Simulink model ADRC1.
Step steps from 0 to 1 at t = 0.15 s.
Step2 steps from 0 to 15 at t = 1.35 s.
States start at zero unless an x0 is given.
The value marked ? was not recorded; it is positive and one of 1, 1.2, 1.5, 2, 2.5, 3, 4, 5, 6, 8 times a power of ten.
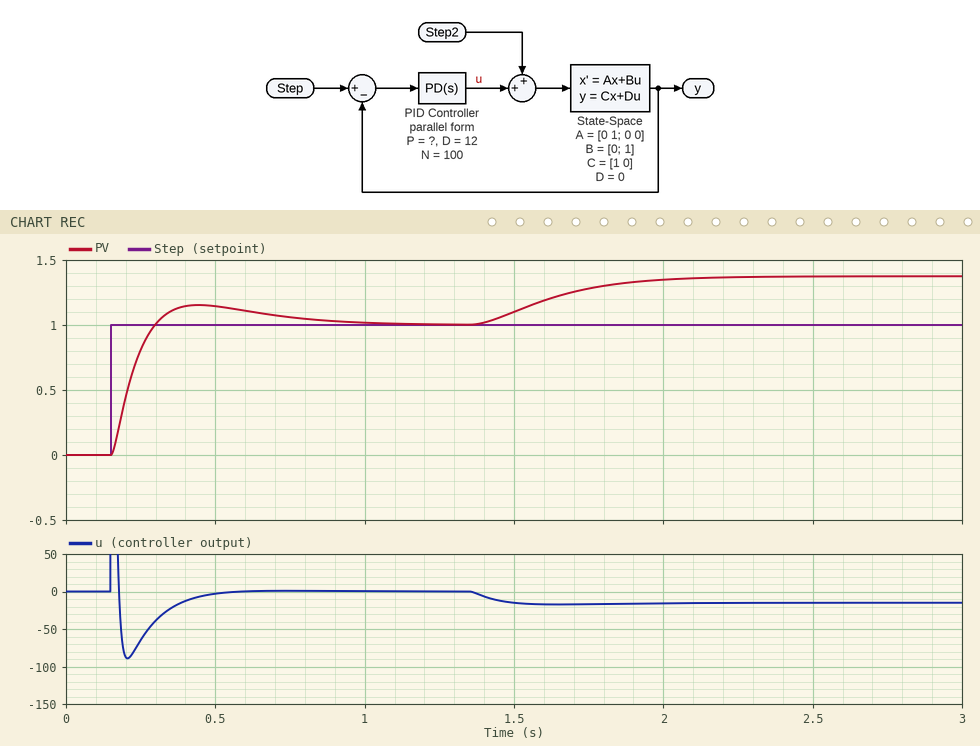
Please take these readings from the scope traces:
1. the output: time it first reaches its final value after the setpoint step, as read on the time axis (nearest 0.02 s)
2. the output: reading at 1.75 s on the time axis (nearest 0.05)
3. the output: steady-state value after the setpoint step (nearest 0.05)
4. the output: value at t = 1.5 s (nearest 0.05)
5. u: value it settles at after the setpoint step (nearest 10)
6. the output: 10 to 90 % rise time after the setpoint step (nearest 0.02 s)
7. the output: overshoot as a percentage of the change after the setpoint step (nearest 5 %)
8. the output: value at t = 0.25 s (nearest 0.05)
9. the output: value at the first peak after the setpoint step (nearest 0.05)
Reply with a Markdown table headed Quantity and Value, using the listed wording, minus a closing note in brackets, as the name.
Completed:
| Quantity | Value |
|---|---|
| the output: time it first reaches its final value after the setpoint step, as read on the time axis | 0.30 s |
| the output: reading at 1.75 s on the time axis | 1.30 |
| the output: steady-state value after the setpoint step | 1.00 |
| the output: value at t = 1.5 s | 1.10 |
| u: value it settles at after the setpoint step | 0 |
| the output: 10 to 90 % rise time after the setpoint step | 0.10 s |
| the output: overshoot as a percentage of the change after the setpoint step | 15 % |
| the output: value at t = 0.25 s | 0.80 |
| the output: value at the first peak after the setpoint step | 1.15 |
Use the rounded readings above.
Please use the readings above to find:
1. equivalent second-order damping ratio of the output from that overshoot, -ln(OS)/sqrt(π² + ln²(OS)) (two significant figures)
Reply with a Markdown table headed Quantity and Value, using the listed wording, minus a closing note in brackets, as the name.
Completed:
| Quantity | Value |
|---|---|
| equivalent second-order damping ratio of the output from that overshoot, -ln(OS)/sqrt(π² + ln²(OS)) | 0.52 |
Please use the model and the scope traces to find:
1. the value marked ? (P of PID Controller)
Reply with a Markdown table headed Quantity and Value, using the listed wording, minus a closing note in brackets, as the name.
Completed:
| Quantity | Value |
|---|---|
| the value marked ? | 40 |
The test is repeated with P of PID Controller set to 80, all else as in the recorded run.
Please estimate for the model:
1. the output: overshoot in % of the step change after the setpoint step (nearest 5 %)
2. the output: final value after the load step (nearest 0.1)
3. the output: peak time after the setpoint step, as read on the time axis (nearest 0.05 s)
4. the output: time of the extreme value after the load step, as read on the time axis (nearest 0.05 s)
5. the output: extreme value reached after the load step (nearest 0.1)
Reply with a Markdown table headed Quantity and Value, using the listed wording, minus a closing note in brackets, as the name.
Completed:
| Quantity | Value |
|---|---|
| the output: overshoot in % of the step change after the setpoint step | 25 % |
| the output: final value after the load step | 1.2 |
| the output: peak time after the setpoint step, as read on the time axis | 0.40 s |
| the output: time of the extreme value after the load step, as read on the time axis | 1.80 s |
| the output: extreme value reached after the load step | 1.2 |
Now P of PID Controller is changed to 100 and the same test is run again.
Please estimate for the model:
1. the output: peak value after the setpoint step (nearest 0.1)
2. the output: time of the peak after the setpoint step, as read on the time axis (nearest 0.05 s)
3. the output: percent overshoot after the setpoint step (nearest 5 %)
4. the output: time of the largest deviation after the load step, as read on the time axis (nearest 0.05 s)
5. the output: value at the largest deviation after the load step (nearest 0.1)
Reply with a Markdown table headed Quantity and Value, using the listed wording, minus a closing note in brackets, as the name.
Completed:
| Quantity | Value |
|---|---|
| the output: peak value after the setpoint step | 1.3 |
| the output: time of the peak after the setpoint step, as read on the time axis | 0.35 s |
| the output: percent overshoot after the setpoint step | 25 % |
| the output: time of the largest deviation after the load step, as read on the time axis | 1.75 s |
| the output: value at the largest deviation after the load step | 1.2 |
